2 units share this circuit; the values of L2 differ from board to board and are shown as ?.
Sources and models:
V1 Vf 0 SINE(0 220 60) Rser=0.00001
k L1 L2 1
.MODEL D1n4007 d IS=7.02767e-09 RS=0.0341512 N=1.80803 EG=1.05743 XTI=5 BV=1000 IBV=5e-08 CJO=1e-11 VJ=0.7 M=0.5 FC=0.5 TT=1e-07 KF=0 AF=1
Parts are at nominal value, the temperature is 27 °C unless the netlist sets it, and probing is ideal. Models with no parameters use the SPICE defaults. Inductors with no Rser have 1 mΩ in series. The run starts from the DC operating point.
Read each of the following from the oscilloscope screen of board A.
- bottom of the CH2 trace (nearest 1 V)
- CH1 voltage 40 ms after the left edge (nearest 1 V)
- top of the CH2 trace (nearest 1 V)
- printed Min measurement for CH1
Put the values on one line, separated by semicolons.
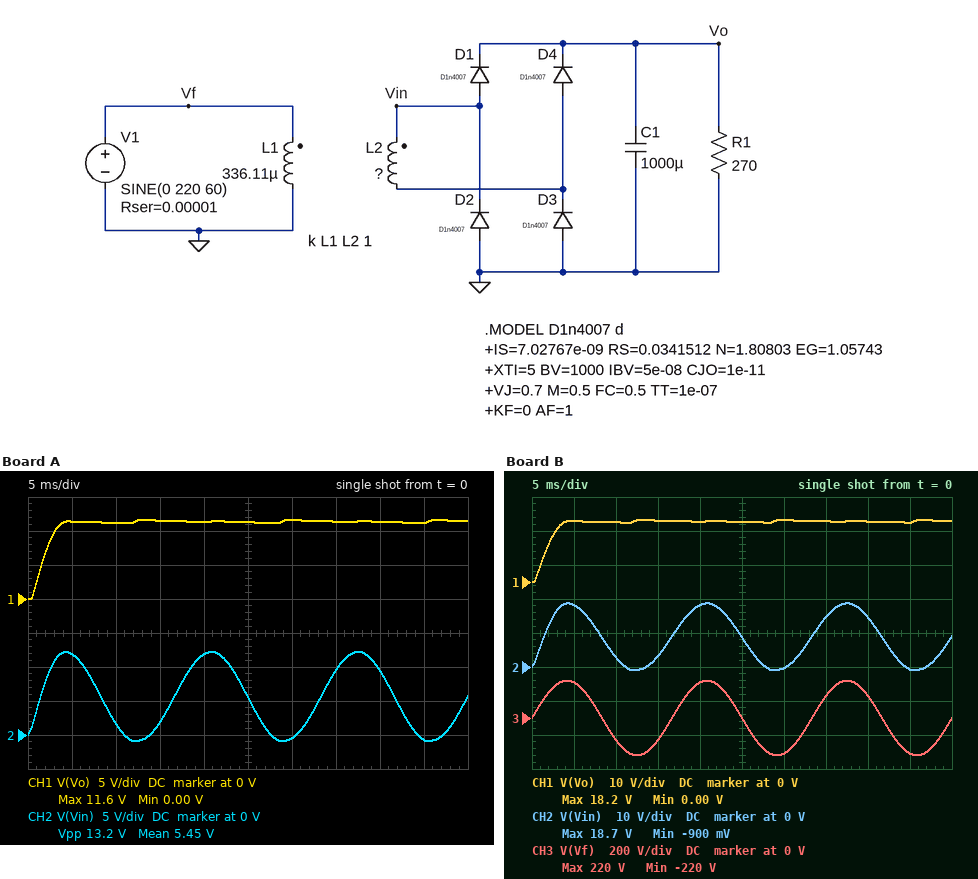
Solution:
-1 V; 11 V; 12 V; 0.00 V
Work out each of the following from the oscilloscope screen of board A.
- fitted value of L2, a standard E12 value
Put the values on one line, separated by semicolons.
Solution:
1.2 µH
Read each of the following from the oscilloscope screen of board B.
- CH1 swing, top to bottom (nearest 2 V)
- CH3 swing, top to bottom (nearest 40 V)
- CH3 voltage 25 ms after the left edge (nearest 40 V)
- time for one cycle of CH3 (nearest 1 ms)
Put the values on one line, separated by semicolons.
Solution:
18 V; 440 V; 0 V; 17 ms
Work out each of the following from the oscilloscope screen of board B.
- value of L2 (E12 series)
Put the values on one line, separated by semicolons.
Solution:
2.7 µH
